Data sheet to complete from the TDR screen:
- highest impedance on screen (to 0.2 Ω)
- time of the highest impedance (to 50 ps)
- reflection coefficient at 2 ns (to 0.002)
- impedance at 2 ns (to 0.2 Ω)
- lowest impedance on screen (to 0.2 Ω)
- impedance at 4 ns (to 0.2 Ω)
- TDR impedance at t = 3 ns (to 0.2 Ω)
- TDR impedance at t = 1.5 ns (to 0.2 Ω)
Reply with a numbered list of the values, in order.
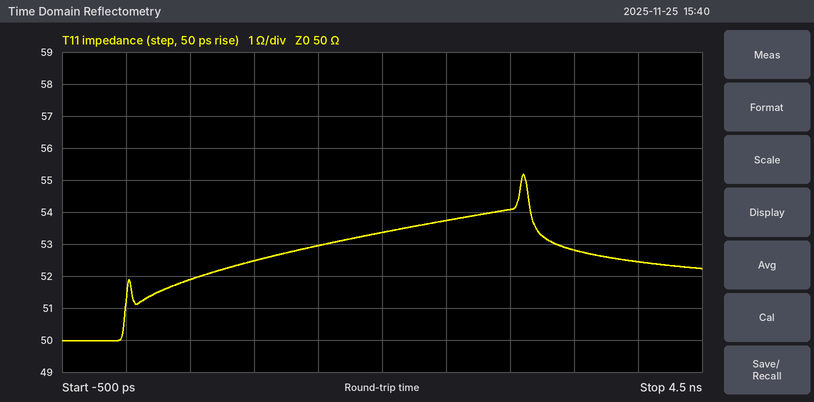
1. 55.2 Ω
2. 3.10 ns
3. +0.032
4. 53.4 Ω
5. 50.0 Ω
6. 52.4 Ω
7. 54.0 Ω
8. 53.0 Ω
